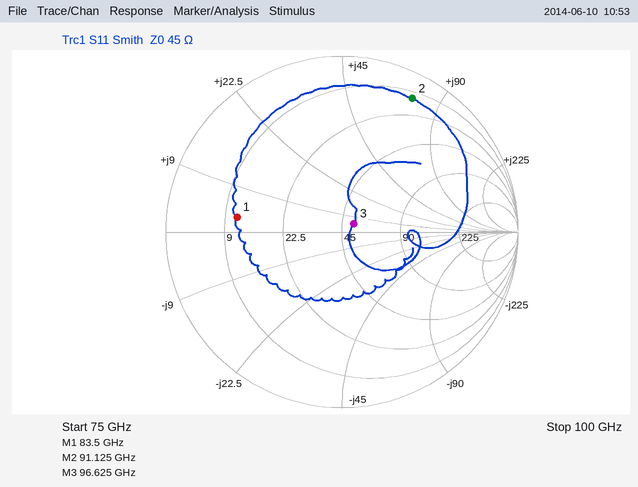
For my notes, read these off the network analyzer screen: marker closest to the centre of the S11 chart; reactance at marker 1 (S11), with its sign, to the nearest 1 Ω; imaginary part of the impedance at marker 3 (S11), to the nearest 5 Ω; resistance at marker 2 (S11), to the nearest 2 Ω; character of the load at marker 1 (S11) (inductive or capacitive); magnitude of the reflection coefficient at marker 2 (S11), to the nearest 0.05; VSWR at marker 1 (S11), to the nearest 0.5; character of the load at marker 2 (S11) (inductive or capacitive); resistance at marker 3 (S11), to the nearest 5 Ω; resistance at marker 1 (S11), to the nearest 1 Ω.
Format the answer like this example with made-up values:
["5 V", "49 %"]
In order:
["marker 3", "+3 Ω", "+5 Ω", "12 Ω", "inductive", "0.85", "4.0", "inductive", "50 Ω", "11 Ω"]
